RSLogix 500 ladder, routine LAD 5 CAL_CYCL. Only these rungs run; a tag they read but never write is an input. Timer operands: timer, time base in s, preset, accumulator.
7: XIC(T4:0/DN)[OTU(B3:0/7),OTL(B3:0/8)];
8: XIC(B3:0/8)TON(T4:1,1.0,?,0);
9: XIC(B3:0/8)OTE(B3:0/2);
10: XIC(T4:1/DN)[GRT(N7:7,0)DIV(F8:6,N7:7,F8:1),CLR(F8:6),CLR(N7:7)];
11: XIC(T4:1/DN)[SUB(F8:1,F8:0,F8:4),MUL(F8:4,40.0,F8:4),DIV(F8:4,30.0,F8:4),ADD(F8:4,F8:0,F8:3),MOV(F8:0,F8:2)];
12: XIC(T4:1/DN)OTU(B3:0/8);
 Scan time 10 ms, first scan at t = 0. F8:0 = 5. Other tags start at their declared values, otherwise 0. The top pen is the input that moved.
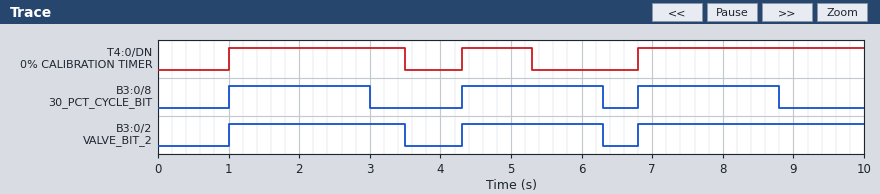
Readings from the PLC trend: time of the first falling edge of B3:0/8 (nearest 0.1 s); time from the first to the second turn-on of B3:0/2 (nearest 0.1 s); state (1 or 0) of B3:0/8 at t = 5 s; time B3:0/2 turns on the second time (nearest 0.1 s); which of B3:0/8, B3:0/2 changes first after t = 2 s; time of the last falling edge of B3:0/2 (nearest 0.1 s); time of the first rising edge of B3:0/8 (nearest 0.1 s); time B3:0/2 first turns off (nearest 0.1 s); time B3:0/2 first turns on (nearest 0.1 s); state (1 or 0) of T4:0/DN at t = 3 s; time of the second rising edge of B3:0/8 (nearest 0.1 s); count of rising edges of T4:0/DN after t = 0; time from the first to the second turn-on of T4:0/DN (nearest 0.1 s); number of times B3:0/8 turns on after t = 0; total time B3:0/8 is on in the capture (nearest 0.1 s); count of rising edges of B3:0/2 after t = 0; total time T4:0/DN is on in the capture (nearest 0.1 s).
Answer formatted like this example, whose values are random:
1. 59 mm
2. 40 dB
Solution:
1. 3.0 s
2. 3.3 s
3. 1
4. 4.3 s
5. B3:0/8
6. 6.3 s
7. 1.0 s
8. 3.5 s
9. 1.0 s
10. 1
11. 4.3 s
12. 3
13. 3.3 s
14. 3
15. 6.0 s
16. 3
17. 6.7 s
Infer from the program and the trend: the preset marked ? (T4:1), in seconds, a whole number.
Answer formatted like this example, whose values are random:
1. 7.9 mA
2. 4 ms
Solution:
1. 2 s
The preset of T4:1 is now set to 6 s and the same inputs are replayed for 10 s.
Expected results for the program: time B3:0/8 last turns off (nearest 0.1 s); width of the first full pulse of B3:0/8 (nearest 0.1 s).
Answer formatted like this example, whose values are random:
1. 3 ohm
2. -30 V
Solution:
1. 7.0 s
2. 6.0 s
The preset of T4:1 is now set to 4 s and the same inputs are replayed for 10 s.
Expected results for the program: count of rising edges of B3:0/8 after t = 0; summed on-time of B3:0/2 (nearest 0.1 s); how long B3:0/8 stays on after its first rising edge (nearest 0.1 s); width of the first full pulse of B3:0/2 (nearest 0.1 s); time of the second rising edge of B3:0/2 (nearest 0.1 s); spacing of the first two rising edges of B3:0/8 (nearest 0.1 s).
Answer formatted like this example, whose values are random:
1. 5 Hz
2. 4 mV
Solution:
1. 2
2. 7.5 s
3. 4.0 s
4. 4.3 s
5. 6.8 s
6. 5.8 s
